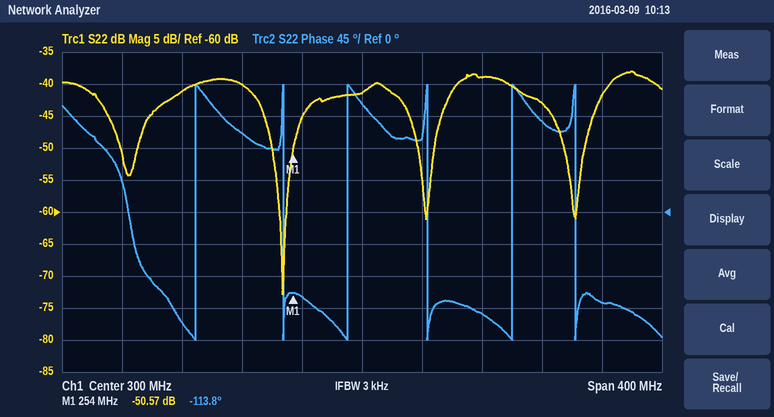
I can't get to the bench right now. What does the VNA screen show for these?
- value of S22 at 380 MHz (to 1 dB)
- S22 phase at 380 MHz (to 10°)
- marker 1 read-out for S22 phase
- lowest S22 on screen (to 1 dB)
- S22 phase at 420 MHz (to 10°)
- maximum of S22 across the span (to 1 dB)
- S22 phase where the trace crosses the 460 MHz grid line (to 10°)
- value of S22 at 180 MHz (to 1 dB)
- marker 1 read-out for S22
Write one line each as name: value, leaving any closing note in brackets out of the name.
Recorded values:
value of S22 at 380 MHz: -39 dB
S22 phase at 380 MHz: -140°
marker 1 read-out for S22 phase: -113.8°
lowest S22 on screen: -73 dB
S22 phase at 420 MHz: 130°
maximum of S22 across the span: -38 dB
S22 phase where the trace crosses the 460 MHz grid line: -130°
value of S22 at 180 MHz: -41 dB
marker 1 read-out for S22: -50.57 dB
